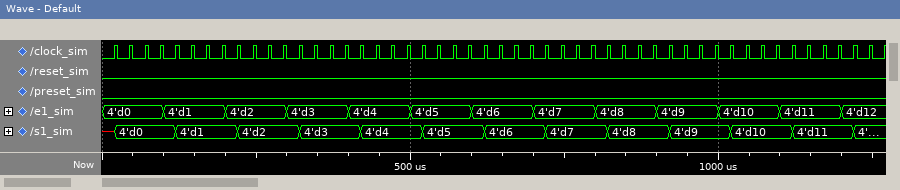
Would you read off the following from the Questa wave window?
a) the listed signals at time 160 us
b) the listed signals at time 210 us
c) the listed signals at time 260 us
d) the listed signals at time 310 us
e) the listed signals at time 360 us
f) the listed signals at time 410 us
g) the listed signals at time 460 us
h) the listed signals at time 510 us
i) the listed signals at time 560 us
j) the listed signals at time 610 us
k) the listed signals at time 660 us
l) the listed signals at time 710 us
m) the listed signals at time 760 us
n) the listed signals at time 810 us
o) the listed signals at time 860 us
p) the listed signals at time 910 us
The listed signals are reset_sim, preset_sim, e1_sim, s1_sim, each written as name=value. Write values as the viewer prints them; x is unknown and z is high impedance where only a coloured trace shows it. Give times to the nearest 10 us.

reset_sim=0, preset_sim=0, e1_sim=4'd1, s1_sim=4'd1
reset_sim=0, preset_sim=0, e1_sim=4'd2, s1_sim=4'd1
reset_sim=0, preset_sim=0, e1_sim=4'd2, s1_sim=4'd2
reset_sim=0, preset_sim=0, e1_sim=4'd3, s1_sim=4'd2
reset_sim=0, preset_sim=0, e1_sim=4'd3, s1_sim=4'd3
reset_sim=0, preset_sim=0, e1_sim=4'd4, s1_sim=4'd3
reset_sim=0, preset_sim=0, e1_sim=4'd4, s1_sim=4'd4
reset_sim=0, preset_sim=0, e1_sim=4'd5, s1_sim=4'd4
reset_sim=0, preset_sim=0, e1_sim=4'd5, s1_sim=4'd5
reset_sim=0, preset_sim=0, e1_sim=4'd6, s1_sim=4'd5
reset_sim=0, preset_sim=0, e1_sim=4'd6, s1_sim=4'd6
reset_sim=0, preset_sim=0, e1_sim=4'd7, s1_sim=4'd6
reset_sim=0, preset_sim=0, e1_sim=4'd7, s1_sim=4'd7
reset_sim=0, preset_sim=0, e1_sim=4'd8, s1_sim=4'd7
reset_sim=0, preset_sim=0, e1_sim=4'd8, s1_sim=4'd8
reset_sim=0, preset_sim=0, e1_sim=4'd9, s1_sim=4'd8
